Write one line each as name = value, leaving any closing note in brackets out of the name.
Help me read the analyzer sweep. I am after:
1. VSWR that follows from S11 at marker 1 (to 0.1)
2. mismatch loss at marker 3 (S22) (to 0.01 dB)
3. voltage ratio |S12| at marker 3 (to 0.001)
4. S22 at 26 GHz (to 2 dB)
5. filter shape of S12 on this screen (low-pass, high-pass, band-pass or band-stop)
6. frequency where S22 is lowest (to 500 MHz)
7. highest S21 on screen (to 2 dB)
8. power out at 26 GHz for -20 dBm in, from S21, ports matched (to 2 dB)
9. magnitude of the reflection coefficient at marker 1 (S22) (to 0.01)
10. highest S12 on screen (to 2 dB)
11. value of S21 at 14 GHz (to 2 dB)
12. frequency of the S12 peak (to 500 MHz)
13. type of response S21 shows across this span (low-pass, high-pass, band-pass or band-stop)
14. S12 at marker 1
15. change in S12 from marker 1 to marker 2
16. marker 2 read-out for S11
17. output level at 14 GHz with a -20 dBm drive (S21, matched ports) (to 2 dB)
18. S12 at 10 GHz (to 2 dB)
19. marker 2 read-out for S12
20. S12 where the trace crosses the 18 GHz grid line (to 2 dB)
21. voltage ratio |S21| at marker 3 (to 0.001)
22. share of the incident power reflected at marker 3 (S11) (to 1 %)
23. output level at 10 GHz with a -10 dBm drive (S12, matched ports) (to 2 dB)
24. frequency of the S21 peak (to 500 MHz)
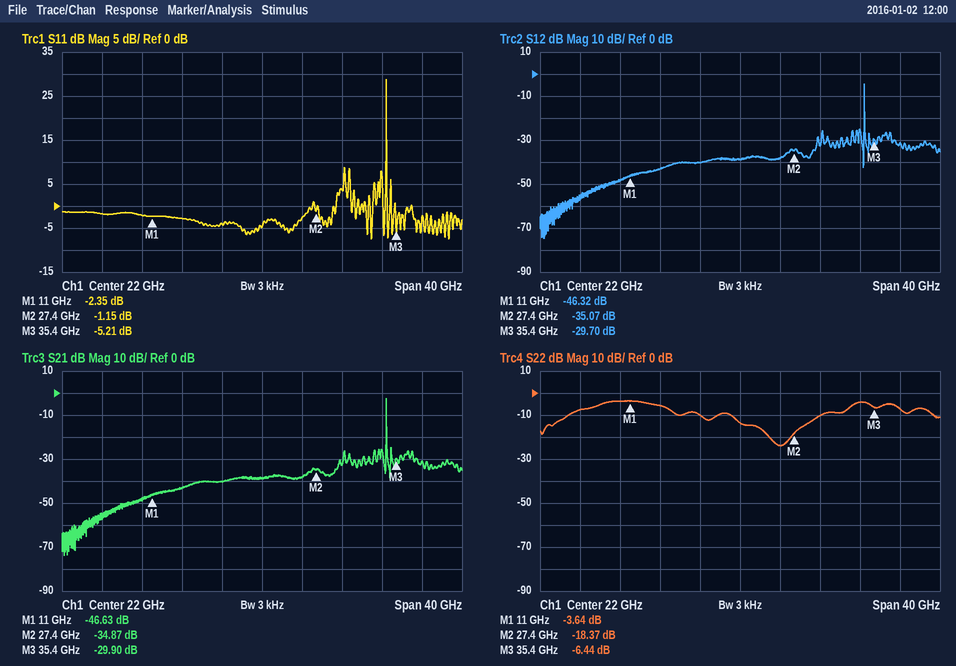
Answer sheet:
VSWR that follows from S11 at marker 1 = 7.4
mismatch loss at marker 3 (S22) = 1.12 dB
voltage ratio |S12| at marker 3 = 0.033
S22 at 26 GHz = -24 dB
filter shape of S12 on this screen = band-pass
frequency where S22 is lowest = 26.0 GHz
highest S21 on screen = -2 dB
power out at 26 GHz for -20 dBm in, from S21, ports matched = -58 dBm
magnitude of the reflection coefficient at marker 1 (S22) = 0.66
highest S12 on screen = -4 dB
value of S21 at 14 GHz = -44 dB
frequency of the S12 peak = 34.5 GHz
type of response S21 shows across this span = band-pass
S12 at marker 1 = -46.32 dB
change in S12 from marker 1 to marker 2 = 11.25 dB
marker 2 read-out for S11 = -1.15 dB
output level at 14 GHz with a -20 dBm drive (S21, matched ports) = -64 dBm
S12 at 10 GHz = -48 dB
marker 2 read-out for S12 = -35.07 dB
S12 where the trace crosses the 18 GHz grid line = -40 dB
voltage ratio |S21| at marker 3 = 0.032
share of the incident power reflected at marker 3 (S11) = 30 %
output level at 10 GHz with a -10 dBm drive (S12, matched ports) = -58 dBm
frequency of the S21 peak = 34.5 GHz
